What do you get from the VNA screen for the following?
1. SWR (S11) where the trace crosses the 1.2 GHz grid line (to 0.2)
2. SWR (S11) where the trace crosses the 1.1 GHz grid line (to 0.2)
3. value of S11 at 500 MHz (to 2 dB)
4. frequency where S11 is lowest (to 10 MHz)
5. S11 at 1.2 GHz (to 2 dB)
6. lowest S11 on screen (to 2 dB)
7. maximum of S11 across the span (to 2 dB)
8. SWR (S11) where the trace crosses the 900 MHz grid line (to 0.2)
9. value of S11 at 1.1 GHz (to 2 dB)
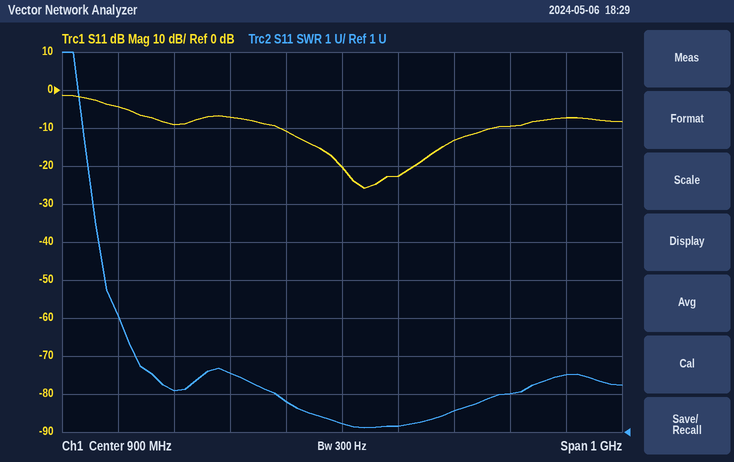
2.0
1.6
-4 dB
940 MHz
-10 dB
-26 dB
-2 dB
1.2
-14 dB
